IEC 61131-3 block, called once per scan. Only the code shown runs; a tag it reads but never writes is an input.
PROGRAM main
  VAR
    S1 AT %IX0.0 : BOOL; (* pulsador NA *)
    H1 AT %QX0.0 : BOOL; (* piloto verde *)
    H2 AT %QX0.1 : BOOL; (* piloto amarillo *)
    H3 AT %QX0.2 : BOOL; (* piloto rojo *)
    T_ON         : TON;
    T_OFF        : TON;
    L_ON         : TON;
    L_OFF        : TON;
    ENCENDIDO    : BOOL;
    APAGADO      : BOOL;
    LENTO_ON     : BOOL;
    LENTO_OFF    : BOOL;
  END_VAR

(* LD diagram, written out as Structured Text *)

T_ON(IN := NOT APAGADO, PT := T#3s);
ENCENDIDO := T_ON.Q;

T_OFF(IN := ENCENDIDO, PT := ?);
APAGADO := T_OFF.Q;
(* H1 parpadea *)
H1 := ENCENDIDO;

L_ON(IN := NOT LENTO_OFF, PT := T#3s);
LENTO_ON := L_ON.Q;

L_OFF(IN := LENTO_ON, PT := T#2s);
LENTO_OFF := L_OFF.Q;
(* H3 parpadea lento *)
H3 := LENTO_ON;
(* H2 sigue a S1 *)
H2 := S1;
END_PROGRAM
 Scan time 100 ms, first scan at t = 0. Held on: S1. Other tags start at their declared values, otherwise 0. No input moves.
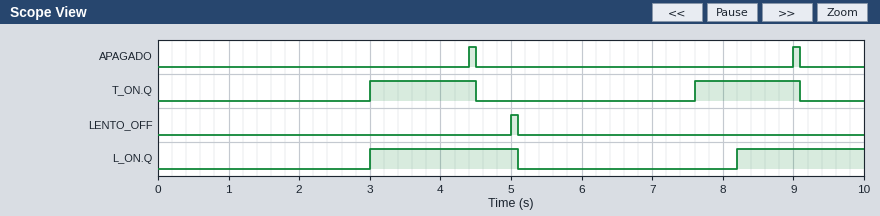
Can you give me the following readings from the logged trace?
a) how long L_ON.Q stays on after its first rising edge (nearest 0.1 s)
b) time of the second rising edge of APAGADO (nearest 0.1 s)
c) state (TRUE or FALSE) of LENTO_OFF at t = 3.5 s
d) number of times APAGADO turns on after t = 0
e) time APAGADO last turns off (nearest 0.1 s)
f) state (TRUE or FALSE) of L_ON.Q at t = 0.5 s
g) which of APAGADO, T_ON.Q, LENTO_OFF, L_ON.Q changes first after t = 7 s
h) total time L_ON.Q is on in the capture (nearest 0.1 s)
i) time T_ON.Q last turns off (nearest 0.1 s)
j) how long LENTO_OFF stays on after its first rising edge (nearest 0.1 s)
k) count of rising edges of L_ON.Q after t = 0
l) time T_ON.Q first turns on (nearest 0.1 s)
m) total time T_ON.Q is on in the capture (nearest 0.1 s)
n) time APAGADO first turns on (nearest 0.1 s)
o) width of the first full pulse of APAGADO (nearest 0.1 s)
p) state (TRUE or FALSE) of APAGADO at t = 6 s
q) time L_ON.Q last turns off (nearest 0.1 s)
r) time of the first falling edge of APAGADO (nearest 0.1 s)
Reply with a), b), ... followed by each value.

a) 2.1 s
b) 9.0 s
c) FALSE
d) 2
e) 9.1 s
f) FALSE
g) T_ON.Q
h) 3.9 s
i) 9.1 s
j) 0.1 s
k) 2
l) 3.0 s
m) 3.0 s
n) 4.4 s
o) 0.1 s
p) FALSE
q) 5.1 s
r) 4.5 s
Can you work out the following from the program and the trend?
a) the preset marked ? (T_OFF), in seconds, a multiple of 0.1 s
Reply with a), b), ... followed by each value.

a) 1.4 s
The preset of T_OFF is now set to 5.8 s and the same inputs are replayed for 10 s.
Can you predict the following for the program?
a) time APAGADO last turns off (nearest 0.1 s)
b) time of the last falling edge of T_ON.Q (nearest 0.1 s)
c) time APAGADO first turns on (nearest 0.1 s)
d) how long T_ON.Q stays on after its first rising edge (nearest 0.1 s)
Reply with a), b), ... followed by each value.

a) 8.9 s
b) 8.9 s
c) 8.8 s
d) 5.9 s
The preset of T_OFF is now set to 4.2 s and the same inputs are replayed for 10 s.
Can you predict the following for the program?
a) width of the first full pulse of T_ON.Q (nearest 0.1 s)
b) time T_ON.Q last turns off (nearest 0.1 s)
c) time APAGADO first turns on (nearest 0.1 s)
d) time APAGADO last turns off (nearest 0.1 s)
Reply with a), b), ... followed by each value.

a) 4.3 s
b) 7.3 s
c) 7.2 s
d) 7.3 s
